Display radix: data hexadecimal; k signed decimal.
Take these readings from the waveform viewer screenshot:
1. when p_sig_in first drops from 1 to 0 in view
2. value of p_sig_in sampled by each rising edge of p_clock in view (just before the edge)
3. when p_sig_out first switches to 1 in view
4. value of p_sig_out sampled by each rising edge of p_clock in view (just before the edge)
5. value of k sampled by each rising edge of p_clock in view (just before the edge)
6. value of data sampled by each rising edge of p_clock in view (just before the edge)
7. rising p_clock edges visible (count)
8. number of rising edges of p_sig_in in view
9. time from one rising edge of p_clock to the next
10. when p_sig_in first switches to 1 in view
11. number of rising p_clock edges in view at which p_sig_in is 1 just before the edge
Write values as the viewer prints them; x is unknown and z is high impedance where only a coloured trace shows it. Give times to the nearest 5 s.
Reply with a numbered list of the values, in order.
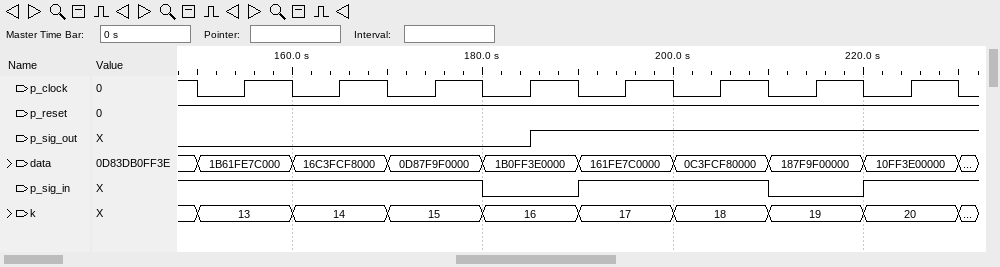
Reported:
1. 180 s
2. 1 1 1 0 1 1 0 1
3. 185 s
4. 0 0 0 0 1 1 1 1
5. 13, 14, 15, 16, 17, 18, 19, 20
6. 1B61FE7C000, 16C3FCF8000, 0D87F9F0000, 1B0FF3E0000, 161FE7C0000, 0C3FCF80000, 187F9F00000, 10FF3E00000
7. 8
8. 2
9. 10 s
10. 190 s
11. 6
